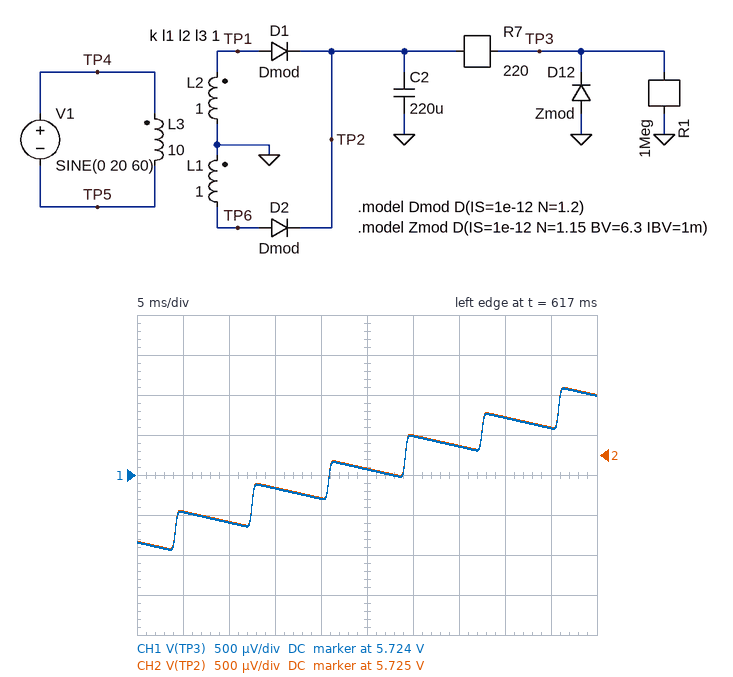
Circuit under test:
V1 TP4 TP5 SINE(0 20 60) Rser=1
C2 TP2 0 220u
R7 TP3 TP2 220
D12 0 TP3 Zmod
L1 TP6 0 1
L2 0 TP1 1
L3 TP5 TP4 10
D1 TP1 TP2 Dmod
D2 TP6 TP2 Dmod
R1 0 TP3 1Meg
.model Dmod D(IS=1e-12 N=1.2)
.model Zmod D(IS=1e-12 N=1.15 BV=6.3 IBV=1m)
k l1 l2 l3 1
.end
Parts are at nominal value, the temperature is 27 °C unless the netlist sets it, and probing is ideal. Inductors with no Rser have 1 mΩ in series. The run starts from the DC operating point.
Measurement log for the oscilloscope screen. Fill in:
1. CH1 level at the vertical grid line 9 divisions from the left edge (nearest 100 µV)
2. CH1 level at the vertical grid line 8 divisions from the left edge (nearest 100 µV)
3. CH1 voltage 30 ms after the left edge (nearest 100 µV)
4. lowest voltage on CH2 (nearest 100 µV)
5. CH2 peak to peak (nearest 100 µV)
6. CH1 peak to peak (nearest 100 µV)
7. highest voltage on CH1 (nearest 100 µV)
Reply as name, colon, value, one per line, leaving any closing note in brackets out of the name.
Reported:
CH1 level at the vertical grid line 9 divisions from the left edge: 5.7241 V
CH1 level at the vertical grid line 8 divisions from the left edge: 5.7242 V
CH1 voltage 30 ms after the left edge: 5.7240 V
lowest voltage on CH2: 5.7238 V
CH2 peak to peak: 2.0 mV
CH1 peak to peak: 2.0 mV
highest voltage on CH1: 5.7246 V
